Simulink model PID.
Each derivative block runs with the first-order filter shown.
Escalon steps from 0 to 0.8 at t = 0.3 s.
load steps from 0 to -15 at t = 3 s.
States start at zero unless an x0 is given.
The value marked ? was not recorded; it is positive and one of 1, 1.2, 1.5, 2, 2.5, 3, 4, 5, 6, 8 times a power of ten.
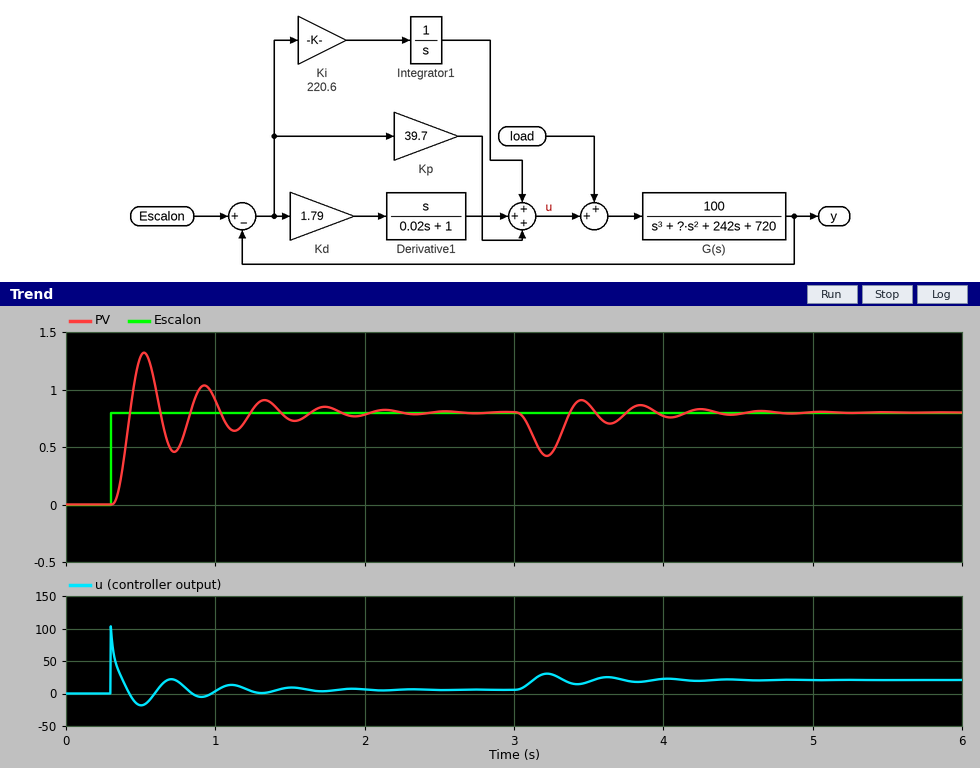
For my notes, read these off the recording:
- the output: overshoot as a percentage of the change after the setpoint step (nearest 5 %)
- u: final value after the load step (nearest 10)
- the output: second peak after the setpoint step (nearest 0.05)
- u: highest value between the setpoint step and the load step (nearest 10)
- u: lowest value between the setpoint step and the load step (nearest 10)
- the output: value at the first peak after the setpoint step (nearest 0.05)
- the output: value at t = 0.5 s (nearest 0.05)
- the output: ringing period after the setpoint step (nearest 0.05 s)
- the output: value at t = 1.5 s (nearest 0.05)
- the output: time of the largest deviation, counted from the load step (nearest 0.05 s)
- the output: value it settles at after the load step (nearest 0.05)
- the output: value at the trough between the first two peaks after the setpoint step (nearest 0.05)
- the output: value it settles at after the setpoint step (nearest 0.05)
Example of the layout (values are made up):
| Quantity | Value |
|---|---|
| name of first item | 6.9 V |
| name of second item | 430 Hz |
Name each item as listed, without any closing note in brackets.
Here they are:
| Quantity | Value |
|---|---|
| the output: overshoot as a percentage of the change after the setpoint step | 65 % |
| u: final value after the load step | 20 |
| the output: second peak after the setpoint step | 1.05 |
| u: highest value between the setpoint step and the load step | 100 |
| u: lowest value between the setpoint step and the load step | -20 |
| the output: value at the first peak after the setpoint step | 1.30 |
| the output: value at t = 0.5 s | 1.30 |
| the output: ringing period after the setpoint step | 0.40 s |
| the output: value at t = 1.5 s | 0.75 |
| the output: time of the largest deviation, counted from the load step | 0.20 s |
| the output: value it settles at after the load step | 0.80 |
| the output: value at the trough between the first two peaks after the setpoint step | 0.45 |
| the output: value it settles at after the setpoint step | 0.80 |
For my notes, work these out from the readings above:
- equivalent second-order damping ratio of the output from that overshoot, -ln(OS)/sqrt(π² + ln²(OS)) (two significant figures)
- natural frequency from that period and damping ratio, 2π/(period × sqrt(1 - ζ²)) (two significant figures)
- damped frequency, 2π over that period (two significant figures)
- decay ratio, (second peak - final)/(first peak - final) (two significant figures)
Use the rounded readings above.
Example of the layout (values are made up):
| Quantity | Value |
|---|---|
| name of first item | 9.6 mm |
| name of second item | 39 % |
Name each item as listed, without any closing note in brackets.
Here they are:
| Quantity | Value |
|---|---|
| equivalent second-order damping ratio of the output from that overshoot, -ln(OS)/sqrt(π² + ln²(OS)) | 0.14 |
| natural frequency from that period and damping ratio, 2π/(period × sqrt(1 - ζ²)) | 16 rad/s |
| damped frequency, 2π over that period | 16 rad/s |
| decay ratio, (second peak - final)/(first peak - final) | 0.50 |
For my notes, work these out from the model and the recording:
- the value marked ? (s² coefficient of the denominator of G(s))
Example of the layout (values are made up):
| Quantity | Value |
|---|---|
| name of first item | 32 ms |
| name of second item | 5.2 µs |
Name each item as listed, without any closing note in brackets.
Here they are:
| Quantity | Value |
|---|---|
| the value marked ? (s² coefficient of the denominator of G(s)) | 25 |
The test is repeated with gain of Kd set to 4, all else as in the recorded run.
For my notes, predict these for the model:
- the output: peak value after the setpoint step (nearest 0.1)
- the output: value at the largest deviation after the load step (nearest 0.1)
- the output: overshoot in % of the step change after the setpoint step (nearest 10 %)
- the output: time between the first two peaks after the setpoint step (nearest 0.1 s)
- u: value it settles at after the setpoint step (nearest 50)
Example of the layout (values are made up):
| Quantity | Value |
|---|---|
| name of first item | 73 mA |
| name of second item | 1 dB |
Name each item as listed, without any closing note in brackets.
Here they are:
| Quantity | Value |
|---|---|
| the output: peak value after the setpoint step | 1.2 |
| the output: value at the largest deviation after the load step | 0.5 |
| the output: overshoot in % of the step change after the setpoint step | 50 % |
| the output: time between the first two peaks after the setpoint step | 0.3 s |
| u: value it settles at after the setpoint step | 0 |
